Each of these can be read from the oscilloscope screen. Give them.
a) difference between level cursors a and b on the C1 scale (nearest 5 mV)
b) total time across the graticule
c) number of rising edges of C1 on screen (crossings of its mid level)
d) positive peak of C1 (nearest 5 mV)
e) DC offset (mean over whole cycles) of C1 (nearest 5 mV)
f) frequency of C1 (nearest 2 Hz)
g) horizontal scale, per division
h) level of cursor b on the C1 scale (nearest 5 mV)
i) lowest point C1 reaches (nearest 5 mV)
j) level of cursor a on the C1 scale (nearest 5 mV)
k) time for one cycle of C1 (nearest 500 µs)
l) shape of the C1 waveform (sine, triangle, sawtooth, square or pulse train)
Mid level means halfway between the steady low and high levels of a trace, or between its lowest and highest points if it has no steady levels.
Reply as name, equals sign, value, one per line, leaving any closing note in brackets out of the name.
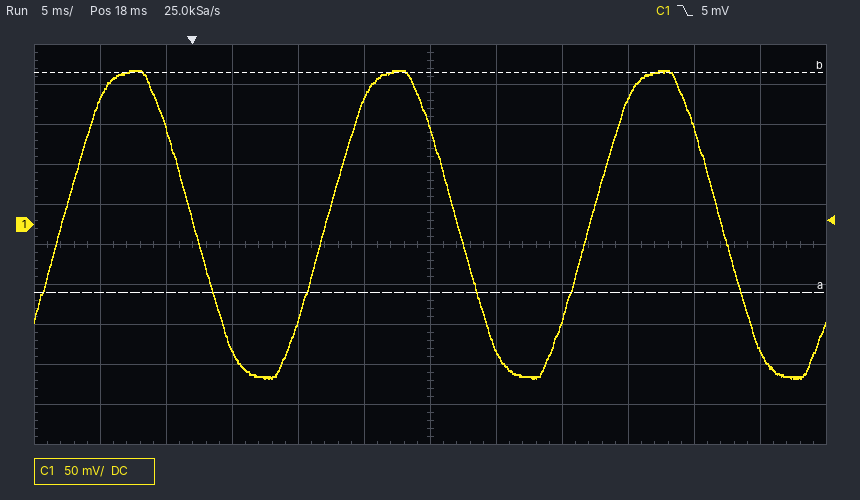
difference between level cursors a and b on the C1 scale = 275 mV
total time across the graticule = 60 ms
number of rising edges of C1 on screen = 3
positive peak of C1 = 190 mV
DC offset (mean over whole cycles) of C1 = 0 mV
frequency of C1 = 50 Hz
horizontal scale, per division = 5 ms
level of cursor b on the C1 scale = 190 mV
lowest point C1 reaches = -190 mV
level of cursor a on the C1 scale = -85 mV
time for one cycle of C1 = 20.0 ms
shape of the C1 waveform = sine
